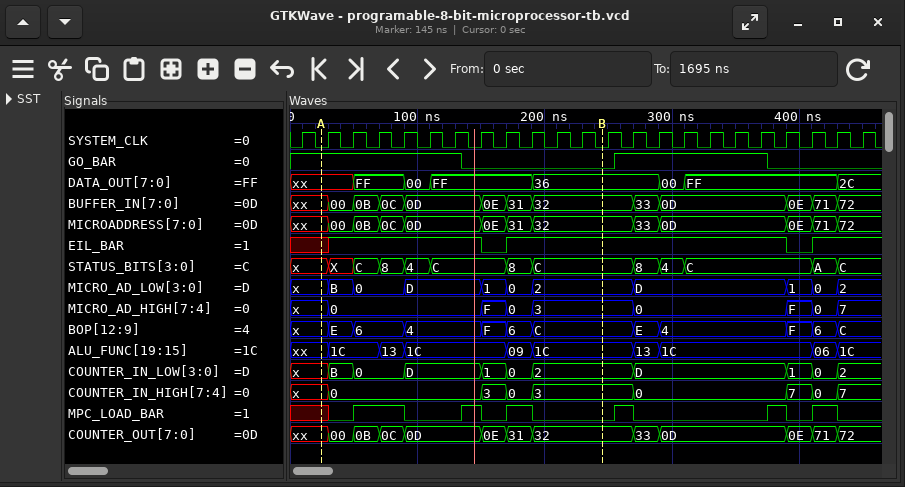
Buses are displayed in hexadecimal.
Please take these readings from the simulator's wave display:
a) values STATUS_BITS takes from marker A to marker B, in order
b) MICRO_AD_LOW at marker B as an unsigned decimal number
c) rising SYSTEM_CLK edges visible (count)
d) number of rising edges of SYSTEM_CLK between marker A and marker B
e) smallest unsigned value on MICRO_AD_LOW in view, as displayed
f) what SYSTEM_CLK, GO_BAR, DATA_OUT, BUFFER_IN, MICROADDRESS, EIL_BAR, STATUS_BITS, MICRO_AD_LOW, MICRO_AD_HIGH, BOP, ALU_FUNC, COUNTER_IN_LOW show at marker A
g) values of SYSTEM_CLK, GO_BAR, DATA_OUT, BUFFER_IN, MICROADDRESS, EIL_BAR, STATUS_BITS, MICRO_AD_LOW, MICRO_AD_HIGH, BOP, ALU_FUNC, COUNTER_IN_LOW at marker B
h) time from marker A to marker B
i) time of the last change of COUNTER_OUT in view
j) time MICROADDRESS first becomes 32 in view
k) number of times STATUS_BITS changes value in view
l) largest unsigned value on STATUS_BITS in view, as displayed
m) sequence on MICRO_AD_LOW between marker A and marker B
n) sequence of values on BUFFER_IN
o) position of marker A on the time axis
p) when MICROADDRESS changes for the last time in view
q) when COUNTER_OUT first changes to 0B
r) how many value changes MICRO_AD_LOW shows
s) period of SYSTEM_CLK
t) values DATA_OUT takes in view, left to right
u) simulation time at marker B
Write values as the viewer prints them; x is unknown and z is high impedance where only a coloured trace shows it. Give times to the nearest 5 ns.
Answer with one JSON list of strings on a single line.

["x, X, C, 8, 4, C, 8, C", "2", "23", "11", "0", "SYSTEM_CLK=0, GO_BAR=1, DATA_OUT=xx, BUFFER_IN=xx, MICROADDRESS=xx, EIL_BAR=x, STATUS_BITS=x, MICRO_AD_LOW=x, MICRO_AD_HIGH=x, BOP=x, ALU_FUNC=xx, COUNTER_IN_LOW=x", "SYSTEM_CLK=0, GO_BAR=0, DATA_OUT=36, BUFFER_IN=32, MICROADDRESS=32, EIL_BAR=1, STATUS_BITS=C, MICRO_AD_LOW=2, MICRO_AD_HIGH=3, BOP=C, ALU_FUNC=1C, COUNTER_IN_LOW=2", "220 ns", "430 ns", "190 ns", "12", "C", "x, B, 0, D, 1, 0, 2", "xx, 00, 0B, 0C, 0D, 0E, 31, 32, 33, 0D, 0E, 71, 72", "25 ns", "430 ns", "50 ns", "10", "20 ns", "xx, FF, 00, FF, 36, 00, FF, 2C", "245 ns"]
